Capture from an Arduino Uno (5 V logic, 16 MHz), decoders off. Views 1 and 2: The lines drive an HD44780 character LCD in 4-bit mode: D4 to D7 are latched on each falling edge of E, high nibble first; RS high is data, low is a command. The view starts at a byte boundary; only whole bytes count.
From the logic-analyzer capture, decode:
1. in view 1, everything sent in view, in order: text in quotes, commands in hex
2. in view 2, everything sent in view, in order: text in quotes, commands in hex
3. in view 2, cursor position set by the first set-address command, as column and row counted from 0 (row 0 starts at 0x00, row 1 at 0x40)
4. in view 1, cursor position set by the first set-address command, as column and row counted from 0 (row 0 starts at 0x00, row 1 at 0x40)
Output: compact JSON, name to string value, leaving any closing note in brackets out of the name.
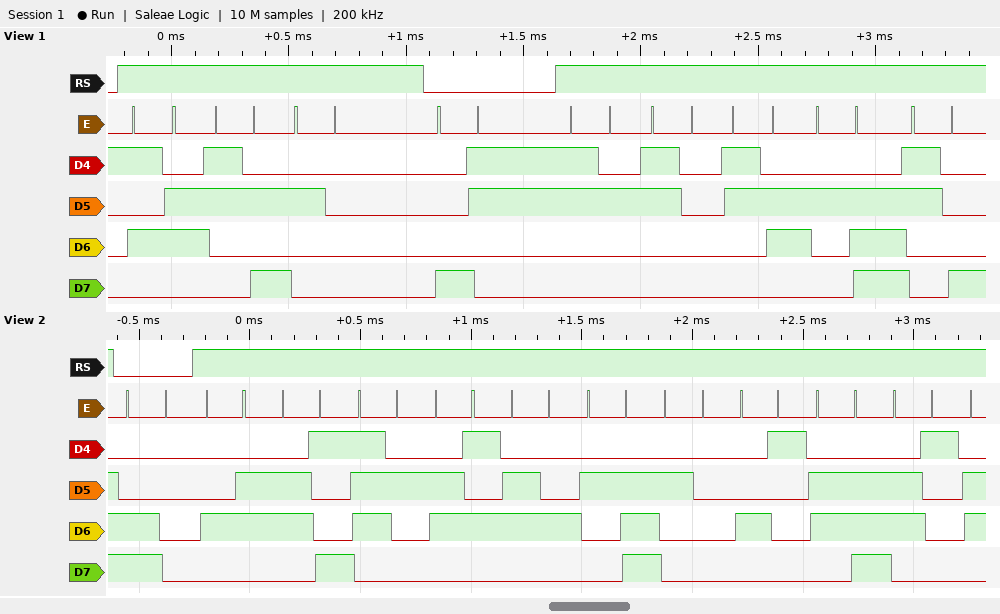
{"in view 1, everything sent in view, in order: text in quotes, commands in hex": "\"V: \" 0x83 \"206.8\"", "in view 2, everything sent in view, in order: text in quotes, commands in hex": "0xC0 \"Fired. Ana\"", "in view 2, cursor position set by the first set-address command, as column and row counted from 0": "column 0, row 1", "in view 1, cursor position set by the first set-address command, as column and row counted from 0": "column 3, row 0"}
